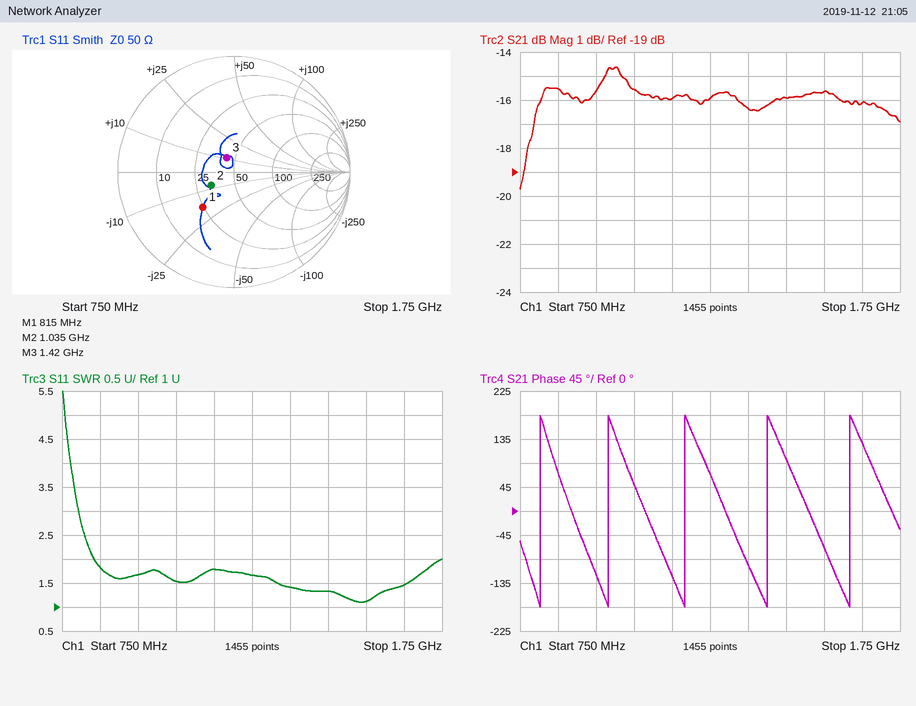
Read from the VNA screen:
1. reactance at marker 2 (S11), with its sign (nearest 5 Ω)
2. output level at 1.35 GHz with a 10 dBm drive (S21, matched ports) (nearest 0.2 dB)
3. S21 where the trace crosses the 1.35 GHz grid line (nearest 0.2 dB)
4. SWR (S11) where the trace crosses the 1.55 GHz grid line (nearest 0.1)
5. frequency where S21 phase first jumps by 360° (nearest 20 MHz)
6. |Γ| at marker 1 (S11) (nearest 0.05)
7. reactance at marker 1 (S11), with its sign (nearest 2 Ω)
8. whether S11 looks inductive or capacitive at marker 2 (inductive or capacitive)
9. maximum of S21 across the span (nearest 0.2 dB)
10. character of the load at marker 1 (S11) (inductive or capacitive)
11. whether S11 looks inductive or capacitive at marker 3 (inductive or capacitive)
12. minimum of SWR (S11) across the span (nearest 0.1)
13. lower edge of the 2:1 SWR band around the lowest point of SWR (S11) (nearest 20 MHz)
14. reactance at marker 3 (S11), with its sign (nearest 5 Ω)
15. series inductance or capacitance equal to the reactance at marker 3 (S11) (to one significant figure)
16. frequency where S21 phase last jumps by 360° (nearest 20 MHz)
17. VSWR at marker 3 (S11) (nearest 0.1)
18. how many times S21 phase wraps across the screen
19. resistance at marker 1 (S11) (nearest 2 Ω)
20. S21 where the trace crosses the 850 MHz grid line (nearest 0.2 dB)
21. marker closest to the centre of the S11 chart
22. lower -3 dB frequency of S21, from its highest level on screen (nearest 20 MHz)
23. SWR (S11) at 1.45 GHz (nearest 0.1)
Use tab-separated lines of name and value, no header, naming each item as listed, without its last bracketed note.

reactance at marker 2 (S11), with its sign	-10 Ω
output level at 1.35 GHz with a 10 dBm drive (S21, matched ports)	-6.4 dBm
S21 where the trace crosses the 1.35 GHz grid line	-16.4 dB
SWR (S11) where the trace crosses the 1.55 GHz grid line	1.1
frequency where S21 phase first jumps by 360°	800 MHz
|Γ| at marker 1 (S11)	0.40
reactance at marker 1 (S11), with its sign	-18 Ω
whether S11 looks inductive or capacitive at marker 2	capacitive
maximum of S21 across the span	-14.6 dB
character of the load at marker 1 (S11)	capacitive
whether S11 looks inductive or capacitive at marker 3	inductive
minimum of SWR (S11) across the span	1.1
lower edge of the 2:1 SWR band around the lowest point of SWR (S11)	840 MHz
reactance at marker 3 (S11), with its sign	+10 Ω
series inductance or capacitance equal to the reactance at marker 3 (S11)	1 nH
frequency where S21 phase last jumps by 360°	1.62 GHz
VSWR at marker 3 (S11)	1.3
how many times S21 phase wraps across the screen	5
resistance at marker 1 (S11)	24 Ω
S21 where the trace crosses the 850 MHz grid line	-15.6 dB
marker closest to the centre of the S11 chart	marker 3
lower -3 dB frequency of S21, from its highest level on screen	780 MHz
SWR (S11) at 1.45 GHz	1.3
